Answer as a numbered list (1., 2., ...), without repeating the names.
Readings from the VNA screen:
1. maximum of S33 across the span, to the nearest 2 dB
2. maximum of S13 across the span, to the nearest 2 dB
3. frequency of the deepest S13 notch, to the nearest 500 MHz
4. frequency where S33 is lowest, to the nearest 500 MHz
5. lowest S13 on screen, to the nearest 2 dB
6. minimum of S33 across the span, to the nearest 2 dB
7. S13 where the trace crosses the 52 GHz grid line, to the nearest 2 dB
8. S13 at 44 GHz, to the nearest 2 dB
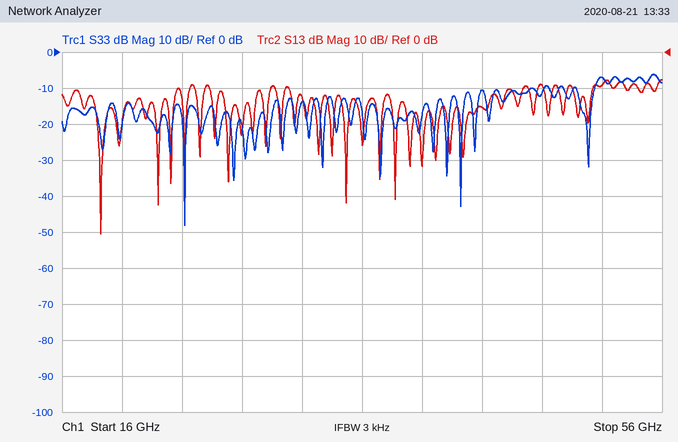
1. -6 dB
2. -8 dB
3. 18.5 GHz
4. 24.0 GHz
5. -50 dB
6. -48 dB
7. -10 dB
8. -16 dB
